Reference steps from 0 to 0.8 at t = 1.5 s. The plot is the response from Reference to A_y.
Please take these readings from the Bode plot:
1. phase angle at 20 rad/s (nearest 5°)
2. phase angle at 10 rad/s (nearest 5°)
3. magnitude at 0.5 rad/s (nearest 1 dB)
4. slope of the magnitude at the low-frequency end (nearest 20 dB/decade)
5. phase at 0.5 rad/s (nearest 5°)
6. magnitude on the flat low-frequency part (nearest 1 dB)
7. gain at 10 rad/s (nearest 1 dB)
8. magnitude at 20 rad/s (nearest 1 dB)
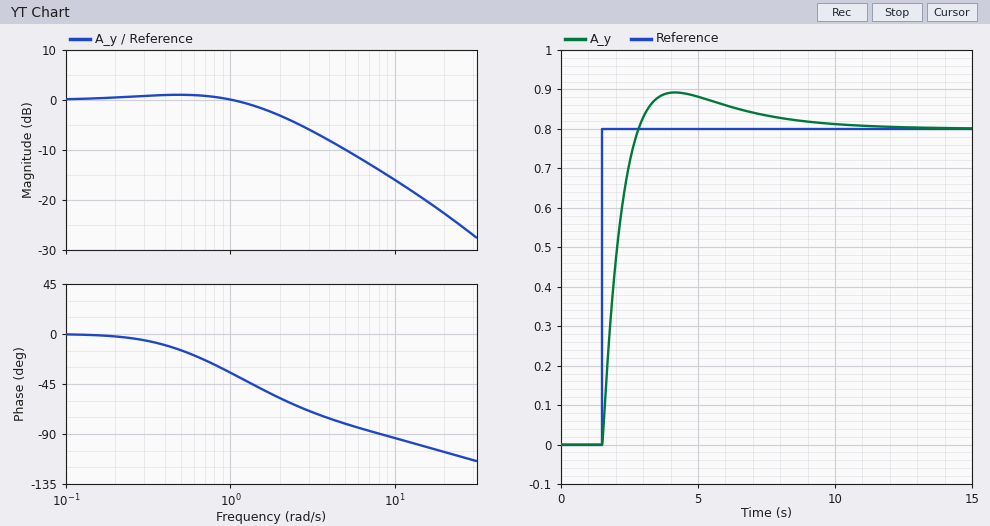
-105°
-95°
1 dB
0 dB/decade
-15°
0 dB
-16 dB
-23 dB
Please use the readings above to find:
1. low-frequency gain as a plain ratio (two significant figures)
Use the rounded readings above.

1.0
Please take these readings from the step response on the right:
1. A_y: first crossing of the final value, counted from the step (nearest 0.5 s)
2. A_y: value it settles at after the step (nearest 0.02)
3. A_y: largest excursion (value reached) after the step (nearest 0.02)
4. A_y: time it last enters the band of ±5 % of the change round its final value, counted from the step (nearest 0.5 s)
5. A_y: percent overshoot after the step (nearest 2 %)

1.5 s
0.80
0.90
5.5 s
12 %
